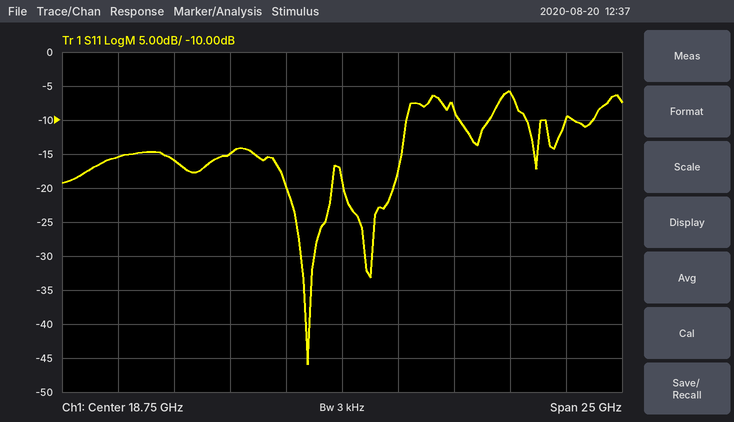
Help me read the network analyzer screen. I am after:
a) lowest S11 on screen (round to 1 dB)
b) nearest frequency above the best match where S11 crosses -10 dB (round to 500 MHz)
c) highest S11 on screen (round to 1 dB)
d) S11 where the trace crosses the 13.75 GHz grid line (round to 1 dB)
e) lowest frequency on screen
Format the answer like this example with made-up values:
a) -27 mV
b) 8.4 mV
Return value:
a) -46 dB
b) 21.5 GHz
c) -6 dB
d) -15 dB
e) 6.25 GHz
